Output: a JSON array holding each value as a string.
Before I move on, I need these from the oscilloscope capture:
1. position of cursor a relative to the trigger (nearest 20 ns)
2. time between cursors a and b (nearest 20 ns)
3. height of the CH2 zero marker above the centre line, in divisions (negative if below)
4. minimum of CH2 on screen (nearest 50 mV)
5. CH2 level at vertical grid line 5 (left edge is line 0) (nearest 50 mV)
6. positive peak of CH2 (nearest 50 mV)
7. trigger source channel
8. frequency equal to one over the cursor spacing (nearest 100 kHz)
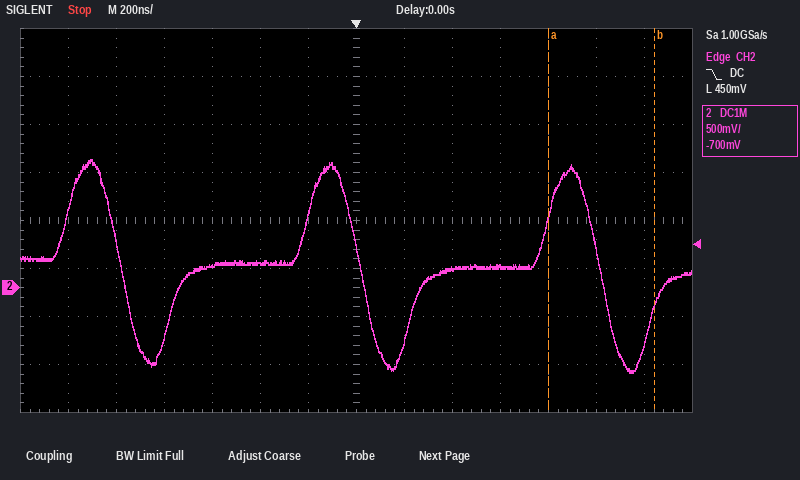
["+800 ns", "440 ns", "-1.4 div", "-900 mV", "250 mV", "1.35 V", "CH2", "2.3 MHz"]
